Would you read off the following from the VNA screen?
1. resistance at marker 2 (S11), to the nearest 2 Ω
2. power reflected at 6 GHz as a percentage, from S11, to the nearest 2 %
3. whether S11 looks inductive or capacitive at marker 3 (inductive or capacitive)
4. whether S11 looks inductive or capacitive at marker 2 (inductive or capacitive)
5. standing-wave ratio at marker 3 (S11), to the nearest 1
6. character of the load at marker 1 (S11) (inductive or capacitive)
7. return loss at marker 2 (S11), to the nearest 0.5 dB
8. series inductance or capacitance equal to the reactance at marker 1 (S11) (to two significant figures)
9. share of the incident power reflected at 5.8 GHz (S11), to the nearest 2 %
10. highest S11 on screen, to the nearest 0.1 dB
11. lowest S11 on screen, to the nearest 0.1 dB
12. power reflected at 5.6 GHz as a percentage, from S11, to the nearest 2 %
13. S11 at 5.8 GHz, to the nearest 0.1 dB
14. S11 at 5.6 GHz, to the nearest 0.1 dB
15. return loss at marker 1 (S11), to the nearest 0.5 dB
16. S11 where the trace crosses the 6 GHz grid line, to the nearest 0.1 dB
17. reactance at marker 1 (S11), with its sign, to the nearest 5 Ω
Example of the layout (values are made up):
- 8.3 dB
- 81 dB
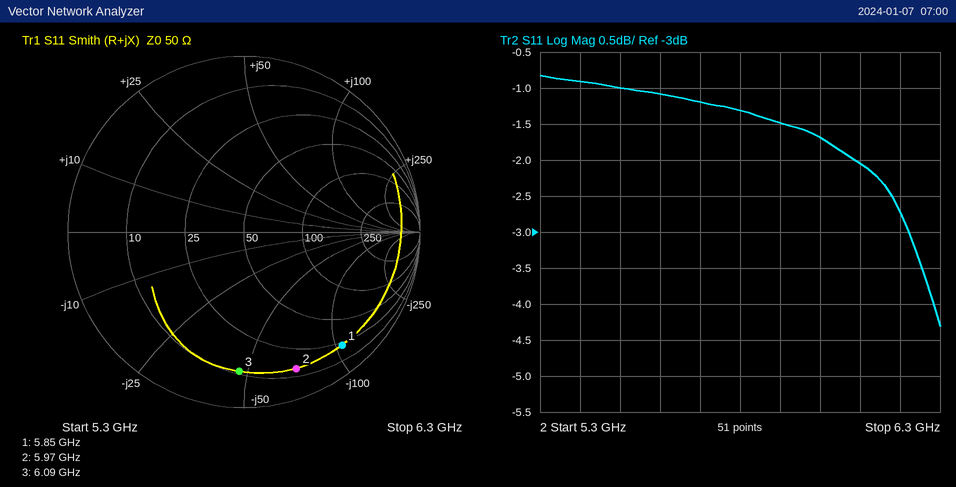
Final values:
- 14 Ω
- 68 %
- capacitive
- capacitive
- 9
- capacitive
- 1.5 dB
- 260 fF
- 74 %
- -0.8 dB
- -4.3 dB
- 78 %
- -1.3 dB
- -1.1 dB
- 1.5 dB
- -1.7 dB
- -105 Ω
